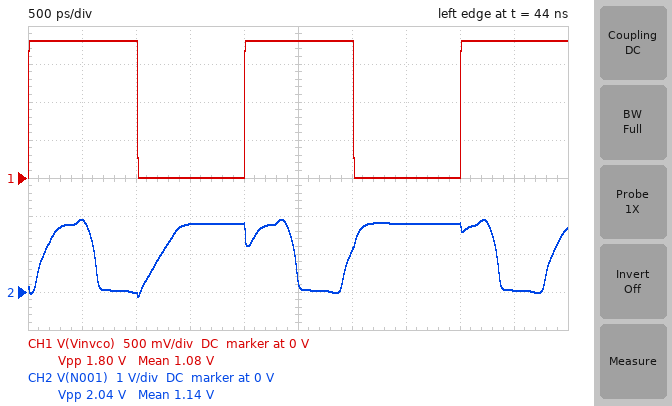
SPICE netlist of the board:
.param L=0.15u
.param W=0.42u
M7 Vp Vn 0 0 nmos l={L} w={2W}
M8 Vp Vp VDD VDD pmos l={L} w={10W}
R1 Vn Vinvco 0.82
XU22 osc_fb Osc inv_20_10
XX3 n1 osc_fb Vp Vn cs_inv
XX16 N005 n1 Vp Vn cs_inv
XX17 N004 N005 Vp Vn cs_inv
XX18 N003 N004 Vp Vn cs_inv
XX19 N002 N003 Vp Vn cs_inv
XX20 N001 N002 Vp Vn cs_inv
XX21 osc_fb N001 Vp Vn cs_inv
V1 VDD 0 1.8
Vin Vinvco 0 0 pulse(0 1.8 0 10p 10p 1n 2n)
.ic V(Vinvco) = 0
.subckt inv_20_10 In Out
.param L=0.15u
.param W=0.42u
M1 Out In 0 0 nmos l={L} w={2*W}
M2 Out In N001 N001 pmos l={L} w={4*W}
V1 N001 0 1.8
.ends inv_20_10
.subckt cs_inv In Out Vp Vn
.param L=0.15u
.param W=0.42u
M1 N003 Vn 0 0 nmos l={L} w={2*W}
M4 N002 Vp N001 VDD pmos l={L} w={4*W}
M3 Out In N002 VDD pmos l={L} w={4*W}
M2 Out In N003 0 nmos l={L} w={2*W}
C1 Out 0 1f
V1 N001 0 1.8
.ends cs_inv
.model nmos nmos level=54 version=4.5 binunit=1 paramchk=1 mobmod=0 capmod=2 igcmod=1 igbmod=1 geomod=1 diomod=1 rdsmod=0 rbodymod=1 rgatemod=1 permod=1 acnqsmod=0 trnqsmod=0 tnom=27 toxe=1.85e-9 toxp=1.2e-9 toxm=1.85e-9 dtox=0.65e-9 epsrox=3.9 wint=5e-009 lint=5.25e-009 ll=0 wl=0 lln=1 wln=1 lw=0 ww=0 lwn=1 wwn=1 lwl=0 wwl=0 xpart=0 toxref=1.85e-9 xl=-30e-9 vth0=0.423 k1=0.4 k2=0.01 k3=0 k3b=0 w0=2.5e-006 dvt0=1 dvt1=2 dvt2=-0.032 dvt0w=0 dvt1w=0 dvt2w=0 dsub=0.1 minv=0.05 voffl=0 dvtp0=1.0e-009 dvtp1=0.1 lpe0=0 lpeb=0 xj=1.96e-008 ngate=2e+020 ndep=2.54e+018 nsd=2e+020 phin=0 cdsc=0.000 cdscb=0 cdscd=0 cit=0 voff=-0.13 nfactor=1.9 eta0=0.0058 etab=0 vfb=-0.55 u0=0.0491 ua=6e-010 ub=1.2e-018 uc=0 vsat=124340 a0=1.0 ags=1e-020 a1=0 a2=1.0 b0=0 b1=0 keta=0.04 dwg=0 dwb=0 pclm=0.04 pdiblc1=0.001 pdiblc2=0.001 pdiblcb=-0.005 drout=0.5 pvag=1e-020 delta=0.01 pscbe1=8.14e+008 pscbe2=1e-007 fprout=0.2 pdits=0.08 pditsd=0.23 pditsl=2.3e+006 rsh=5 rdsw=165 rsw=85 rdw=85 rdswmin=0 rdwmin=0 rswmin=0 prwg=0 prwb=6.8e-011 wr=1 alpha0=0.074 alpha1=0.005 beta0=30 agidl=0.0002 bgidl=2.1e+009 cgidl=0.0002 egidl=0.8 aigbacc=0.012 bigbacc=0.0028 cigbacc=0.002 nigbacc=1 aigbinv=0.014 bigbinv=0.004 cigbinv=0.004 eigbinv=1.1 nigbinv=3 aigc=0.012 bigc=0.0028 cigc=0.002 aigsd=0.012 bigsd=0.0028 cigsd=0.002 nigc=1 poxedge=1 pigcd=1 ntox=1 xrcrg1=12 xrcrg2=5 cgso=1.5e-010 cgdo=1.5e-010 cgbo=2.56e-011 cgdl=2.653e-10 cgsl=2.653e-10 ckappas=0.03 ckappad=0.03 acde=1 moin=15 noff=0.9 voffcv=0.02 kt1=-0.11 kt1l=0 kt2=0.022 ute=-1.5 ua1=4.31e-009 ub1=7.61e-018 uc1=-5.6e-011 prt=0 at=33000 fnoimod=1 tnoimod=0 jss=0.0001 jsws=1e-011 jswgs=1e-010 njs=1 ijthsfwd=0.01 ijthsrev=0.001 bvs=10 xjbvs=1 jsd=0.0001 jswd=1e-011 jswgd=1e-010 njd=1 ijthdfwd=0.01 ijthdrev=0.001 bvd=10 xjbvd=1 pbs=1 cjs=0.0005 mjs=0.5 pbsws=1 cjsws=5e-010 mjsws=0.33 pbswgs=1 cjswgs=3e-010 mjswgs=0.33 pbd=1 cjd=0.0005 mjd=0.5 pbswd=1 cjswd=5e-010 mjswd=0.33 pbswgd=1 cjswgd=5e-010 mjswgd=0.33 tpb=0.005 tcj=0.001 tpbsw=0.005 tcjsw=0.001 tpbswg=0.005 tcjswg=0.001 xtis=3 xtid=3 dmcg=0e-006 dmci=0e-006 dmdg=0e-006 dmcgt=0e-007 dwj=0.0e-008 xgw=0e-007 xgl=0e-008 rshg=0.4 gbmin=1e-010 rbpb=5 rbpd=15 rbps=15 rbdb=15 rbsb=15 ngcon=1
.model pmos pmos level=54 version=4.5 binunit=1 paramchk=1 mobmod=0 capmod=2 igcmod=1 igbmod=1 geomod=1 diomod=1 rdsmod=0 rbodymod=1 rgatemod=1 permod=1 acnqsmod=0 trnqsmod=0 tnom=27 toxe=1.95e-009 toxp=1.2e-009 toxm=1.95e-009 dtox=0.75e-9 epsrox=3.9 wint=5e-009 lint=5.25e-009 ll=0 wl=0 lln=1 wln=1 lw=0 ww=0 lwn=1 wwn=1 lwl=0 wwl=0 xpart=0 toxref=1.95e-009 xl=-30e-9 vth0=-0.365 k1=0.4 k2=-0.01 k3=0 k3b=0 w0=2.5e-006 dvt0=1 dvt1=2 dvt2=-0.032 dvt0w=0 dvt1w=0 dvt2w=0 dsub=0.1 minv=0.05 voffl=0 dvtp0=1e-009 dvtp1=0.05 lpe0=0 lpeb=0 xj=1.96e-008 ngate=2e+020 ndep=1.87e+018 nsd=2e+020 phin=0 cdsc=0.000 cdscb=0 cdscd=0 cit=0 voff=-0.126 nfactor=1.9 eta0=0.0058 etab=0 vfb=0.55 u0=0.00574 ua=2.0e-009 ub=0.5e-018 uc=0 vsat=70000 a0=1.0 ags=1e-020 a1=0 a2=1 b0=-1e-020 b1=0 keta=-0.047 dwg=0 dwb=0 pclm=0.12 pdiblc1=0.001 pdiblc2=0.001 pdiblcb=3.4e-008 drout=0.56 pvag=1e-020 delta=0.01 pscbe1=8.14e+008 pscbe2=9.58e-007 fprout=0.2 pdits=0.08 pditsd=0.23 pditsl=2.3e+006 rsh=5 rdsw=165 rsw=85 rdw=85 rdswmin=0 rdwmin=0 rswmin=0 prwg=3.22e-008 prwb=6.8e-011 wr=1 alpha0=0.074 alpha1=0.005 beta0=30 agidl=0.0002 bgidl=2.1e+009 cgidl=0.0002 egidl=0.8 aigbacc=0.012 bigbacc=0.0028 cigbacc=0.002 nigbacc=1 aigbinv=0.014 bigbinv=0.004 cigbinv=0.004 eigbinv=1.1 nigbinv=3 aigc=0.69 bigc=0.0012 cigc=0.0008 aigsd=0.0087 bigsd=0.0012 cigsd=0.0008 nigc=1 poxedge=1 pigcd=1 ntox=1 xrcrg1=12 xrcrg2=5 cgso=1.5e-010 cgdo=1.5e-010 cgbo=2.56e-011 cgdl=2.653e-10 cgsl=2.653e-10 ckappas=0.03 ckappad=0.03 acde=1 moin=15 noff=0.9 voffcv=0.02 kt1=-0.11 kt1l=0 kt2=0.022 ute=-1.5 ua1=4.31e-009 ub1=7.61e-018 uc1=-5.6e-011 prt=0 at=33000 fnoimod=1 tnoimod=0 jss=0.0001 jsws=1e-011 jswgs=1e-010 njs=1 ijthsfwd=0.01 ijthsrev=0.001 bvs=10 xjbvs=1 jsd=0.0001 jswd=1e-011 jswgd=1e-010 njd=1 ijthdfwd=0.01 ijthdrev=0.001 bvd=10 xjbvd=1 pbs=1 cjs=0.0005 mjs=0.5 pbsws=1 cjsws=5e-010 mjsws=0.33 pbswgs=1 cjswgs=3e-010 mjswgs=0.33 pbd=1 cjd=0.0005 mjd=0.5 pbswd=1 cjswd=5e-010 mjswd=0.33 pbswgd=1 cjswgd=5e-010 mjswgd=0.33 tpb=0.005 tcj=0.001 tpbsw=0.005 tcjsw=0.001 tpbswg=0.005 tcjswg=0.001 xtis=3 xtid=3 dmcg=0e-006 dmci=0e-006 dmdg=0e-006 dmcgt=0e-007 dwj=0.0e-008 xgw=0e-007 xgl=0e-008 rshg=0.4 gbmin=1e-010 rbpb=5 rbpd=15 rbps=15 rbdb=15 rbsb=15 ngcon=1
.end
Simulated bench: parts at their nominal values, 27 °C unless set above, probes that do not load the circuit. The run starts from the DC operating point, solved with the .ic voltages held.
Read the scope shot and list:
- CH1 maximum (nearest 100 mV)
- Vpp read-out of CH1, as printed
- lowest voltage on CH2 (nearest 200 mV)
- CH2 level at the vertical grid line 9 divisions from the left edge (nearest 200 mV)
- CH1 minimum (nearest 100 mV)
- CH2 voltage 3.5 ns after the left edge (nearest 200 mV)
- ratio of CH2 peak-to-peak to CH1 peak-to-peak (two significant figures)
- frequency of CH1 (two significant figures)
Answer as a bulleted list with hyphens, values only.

- 1.8 V
- 1.80 V
- -200 mV
- 0 V
- 0 V
- 1.8 V
- 1.1
- 500 MHz
